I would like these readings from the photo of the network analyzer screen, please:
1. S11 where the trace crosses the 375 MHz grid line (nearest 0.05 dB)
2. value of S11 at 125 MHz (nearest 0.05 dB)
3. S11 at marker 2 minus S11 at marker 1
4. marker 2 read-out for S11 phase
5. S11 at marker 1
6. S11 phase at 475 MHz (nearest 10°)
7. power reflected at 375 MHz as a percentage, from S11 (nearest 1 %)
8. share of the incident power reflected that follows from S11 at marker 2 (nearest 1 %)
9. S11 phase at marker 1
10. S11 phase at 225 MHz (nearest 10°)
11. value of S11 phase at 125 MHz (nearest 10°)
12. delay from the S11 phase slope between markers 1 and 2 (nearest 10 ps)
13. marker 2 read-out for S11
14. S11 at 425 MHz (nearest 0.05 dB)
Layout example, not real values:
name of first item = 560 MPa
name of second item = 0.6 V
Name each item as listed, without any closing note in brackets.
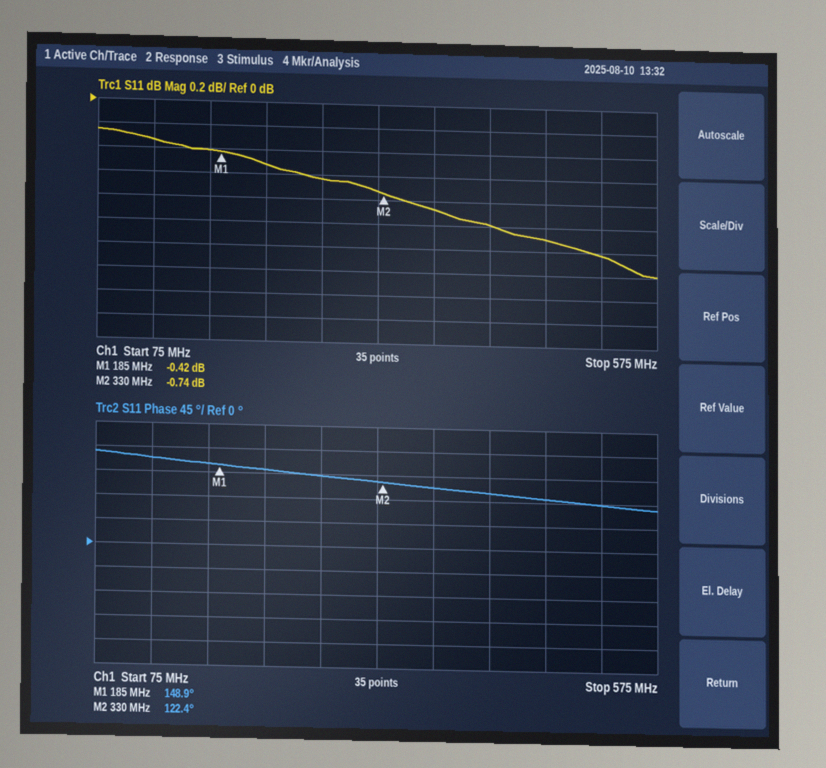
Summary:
S11 where the trace crosses the 375 MHz grid line = -0.85 dB
value of S11 at 125 MHz = -0.35 dB
S11 at marker 2 minus S11 at marker 1 = -0.32 dB
marker 2 read-out for S11 phase = 122.4°
S11 at marker 1 = -0.42 dB
S11 phase at 475 MHz = 100°
power reflected at 375 MHz as a percentage, from S11 = 82 %
share of the incident power reflected that follows from S11 at marker 2 = 84 %
S11 phase at marker 1 = 148.9°
S11 phase at 225 MHz = 140°
value of S11 phase at 125 MHz = 160°
delay from the S11 phase slope between markers 1 and 2 = 510 ps
marker 2 read-out for S11 = -0.74 dB
S11 at 425 MHz = -1.00 dB
